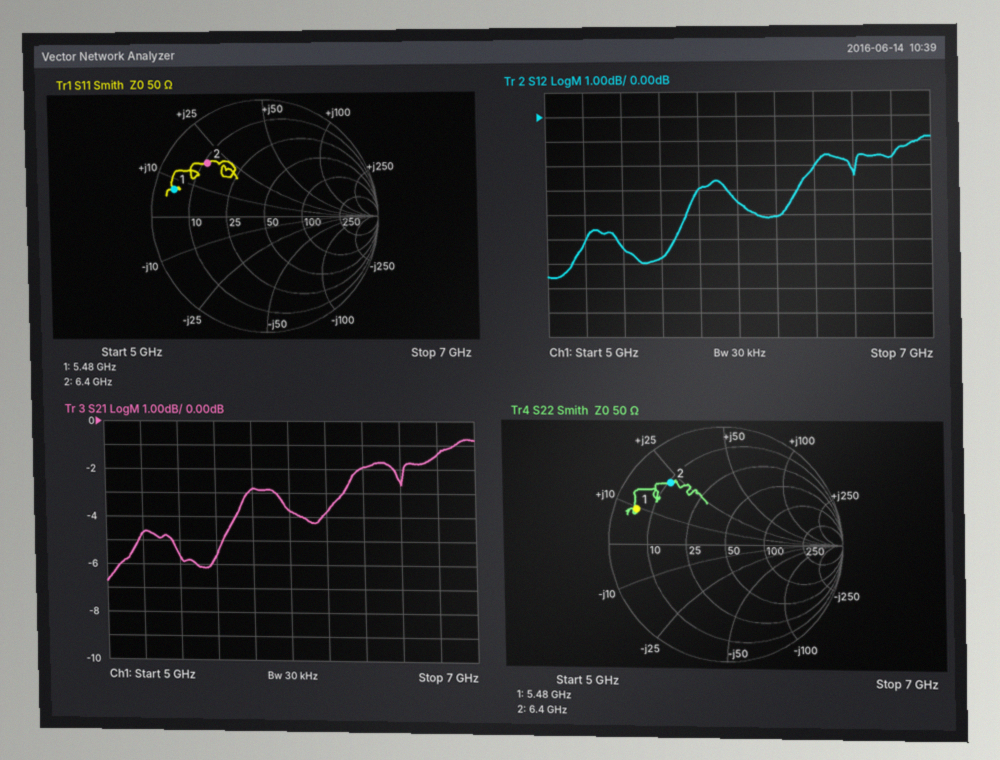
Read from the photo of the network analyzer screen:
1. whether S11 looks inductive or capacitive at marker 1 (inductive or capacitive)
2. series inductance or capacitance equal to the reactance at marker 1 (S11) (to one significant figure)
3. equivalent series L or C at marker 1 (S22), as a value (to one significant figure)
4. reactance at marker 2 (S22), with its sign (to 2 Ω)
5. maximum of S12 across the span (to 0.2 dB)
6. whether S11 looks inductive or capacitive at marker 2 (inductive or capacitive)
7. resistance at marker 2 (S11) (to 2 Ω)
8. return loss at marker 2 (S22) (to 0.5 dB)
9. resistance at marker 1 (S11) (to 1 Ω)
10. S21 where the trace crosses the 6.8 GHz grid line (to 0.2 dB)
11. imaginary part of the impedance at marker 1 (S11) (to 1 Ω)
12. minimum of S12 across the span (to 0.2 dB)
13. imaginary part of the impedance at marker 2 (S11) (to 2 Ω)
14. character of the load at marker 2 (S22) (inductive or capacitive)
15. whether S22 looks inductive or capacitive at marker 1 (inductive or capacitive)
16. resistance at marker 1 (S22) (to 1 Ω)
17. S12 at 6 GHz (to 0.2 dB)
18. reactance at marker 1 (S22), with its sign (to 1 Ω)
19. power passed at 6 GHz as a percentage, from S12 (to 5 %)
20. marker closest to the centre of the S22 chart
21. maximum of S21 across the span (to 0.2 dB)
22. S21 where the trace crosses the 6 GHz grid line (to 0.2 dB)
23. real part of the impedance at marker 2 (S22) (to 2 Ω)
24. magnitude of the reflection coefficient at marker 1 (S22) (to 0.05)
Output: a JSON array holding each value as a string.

["inductive", "200 pH", "300 pH", "+22 Ω", "-0.8 dB", "inductive", "12 Ω", "3.0 dB", "5 Ω", "-1.4 dB", "+7 Ω", "-6.6 dB", "+18 Ω", "inductive", "inductive", "5 Ω", "-3.4 dB", "+9 Ω", "45 %", "marker 2", "-0.8 dB", "-3.8 dB", "10 Ω", "0.80"]
